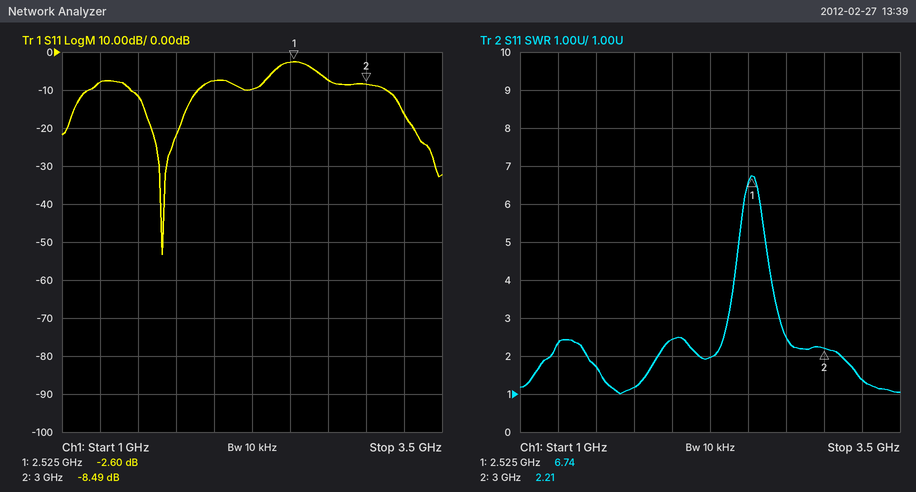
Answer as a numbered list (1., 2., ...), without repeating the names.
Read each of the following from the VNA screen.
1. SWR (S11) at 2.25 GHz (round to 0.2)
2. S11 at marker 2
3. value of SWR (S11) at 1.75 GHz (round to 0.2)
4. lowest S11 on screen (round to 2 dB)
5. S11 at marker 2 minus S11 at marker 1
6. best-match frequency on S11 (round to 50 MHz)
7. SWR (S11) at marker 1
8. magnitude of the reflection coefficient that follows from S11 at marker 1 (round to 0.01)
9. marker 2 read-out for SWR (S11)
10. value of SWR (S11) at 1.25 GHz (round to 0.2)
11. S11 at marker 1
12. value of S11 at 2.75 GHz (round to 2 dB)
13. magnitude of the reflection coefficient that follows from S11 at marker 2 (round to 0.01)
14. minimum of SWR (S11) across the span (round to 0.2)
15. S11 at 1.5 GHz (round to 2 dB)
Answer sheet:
1. 2.0
2. -8.49 dB
3. 1.2
4. -54 dB
5. -5.89 dB
6. 1.65 GHz
7. 6.74
8. 0.74
9. 2.21
10. 2.4
11. -2.60 dB
12. -8 dB
13. 0.38
14. 1.0
15. -12 dB
